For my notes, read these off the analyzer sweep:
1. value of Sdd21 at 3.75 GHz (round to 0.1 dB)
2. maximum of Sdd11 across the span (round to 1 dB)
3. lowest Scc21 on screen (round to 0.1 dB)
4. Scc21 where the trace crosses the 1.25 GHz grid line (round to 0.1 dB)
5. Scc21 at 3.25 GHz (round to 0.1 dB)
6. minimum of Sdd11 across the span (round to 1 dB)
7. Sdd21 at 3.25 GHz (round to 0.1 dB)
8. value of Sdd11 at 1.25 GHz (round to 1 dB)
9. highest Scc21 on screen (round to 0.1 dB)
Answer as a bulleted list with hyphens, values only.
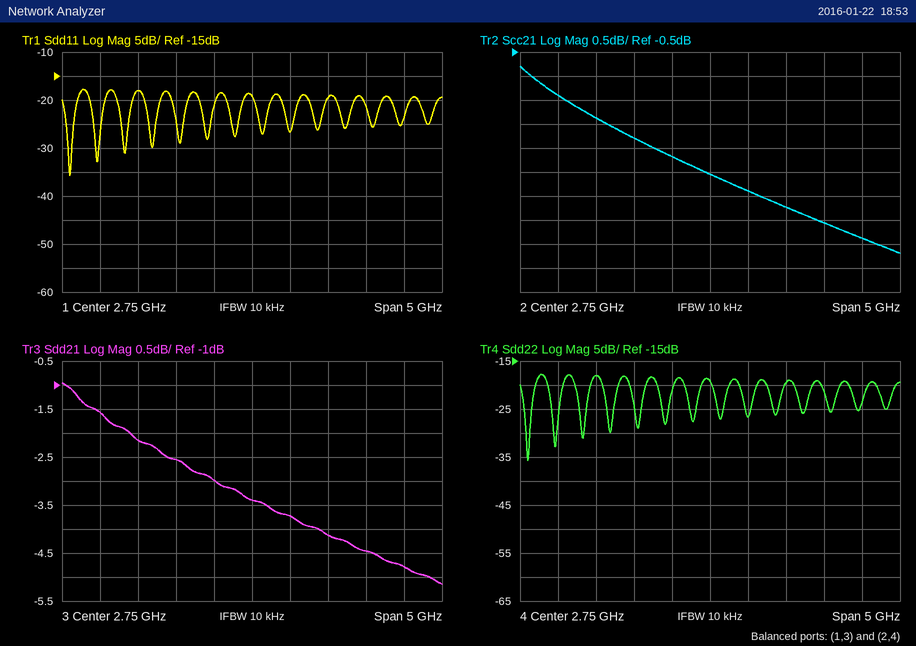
- -4.1 dB
- -18 dB
- -4.7 dB
- -1.9 dB
- -3.4 dB
- -36 dB
- -3.7 dB
- -18 dB
- -0.8 dB
